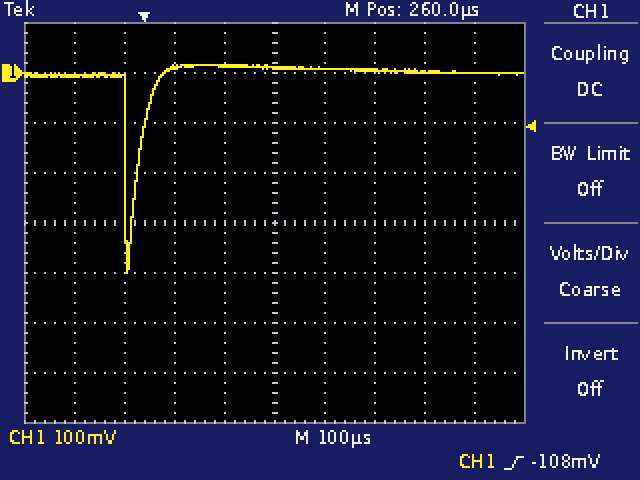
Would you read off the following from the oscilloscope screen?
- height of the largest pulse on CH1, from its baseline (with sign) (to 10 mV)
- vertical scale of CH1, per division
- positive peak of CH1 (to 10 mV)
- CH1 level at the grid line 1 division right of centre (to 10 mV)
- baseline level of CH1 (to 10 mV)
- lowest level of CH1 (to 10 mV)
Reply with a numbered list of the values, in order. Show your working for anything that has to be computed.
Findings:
1. -400 mV − (0 mV) = -400 mV
2. 100 mV
3. 20 mV
4. 10 mV
5. 0 mV
6. -400 mV
